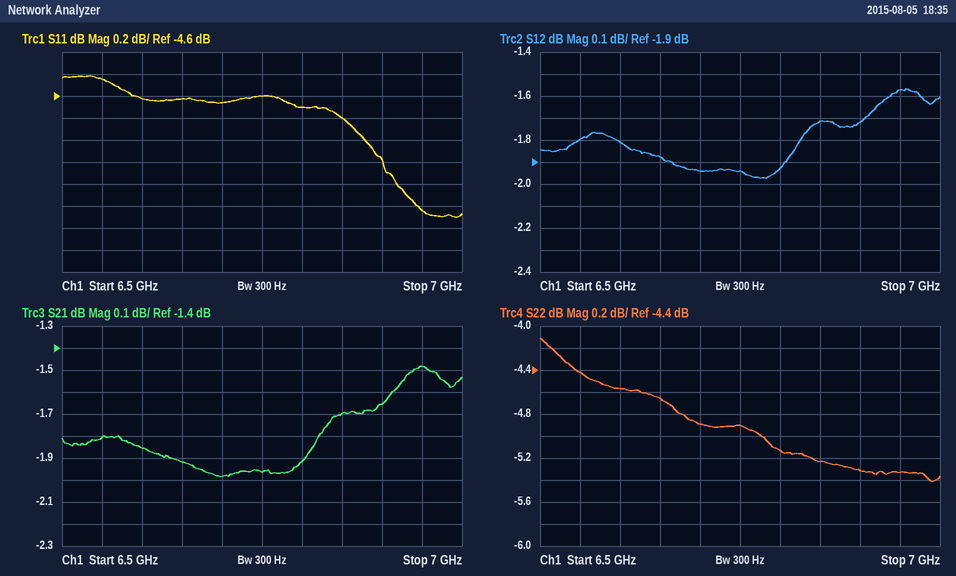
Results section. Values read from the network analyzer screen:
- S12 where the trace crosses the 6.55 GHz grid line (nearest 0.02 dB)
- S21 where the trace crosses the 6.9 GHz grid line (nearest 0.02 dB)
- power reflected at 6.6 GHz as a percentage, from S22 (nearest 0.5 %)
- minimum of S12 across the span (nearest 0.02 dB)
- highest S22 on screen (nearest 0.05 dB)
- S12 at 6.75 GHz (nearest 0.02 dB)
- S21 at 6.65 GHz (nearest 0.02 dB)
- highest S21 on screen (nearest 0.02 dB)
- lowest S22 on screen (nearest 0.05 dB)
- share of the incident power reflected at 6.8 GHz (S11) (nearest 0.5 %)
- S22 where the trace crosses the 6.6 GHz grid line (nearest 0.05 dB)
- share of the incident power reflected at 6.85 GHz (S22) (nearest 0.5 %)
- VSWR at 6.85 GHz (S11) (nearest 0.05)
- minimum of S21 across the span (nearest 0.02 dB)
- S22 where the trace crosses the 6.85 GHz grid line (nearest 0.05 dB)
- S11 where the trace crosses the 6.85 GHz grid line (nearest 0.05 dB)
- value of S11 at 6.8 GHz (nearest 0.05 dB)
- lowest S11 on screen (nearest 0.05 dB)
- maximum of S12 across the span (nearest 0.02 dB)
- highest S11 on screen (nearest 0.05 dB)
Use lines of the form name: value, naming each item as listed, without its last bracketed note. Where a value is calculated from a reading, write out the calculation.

S12 where the trace crosses the 6.55 GHz grid line: -1.80 dB
S21 where the trace crosses the 6.9 GHz grid line: -1.66 dB
power reflected at 6.6 GHz as a percentage, from S22: 10^(-4.55/10) ≈ 35.1 %, so 35.0 % to the nearest 0.5 %
minimum of S12 across the span: -1.98 dB
highest S22 on screen: -4.10 dB
S12 at 6.75 GHz: -1.94 dB
S21 at 6.65 GHz: -1.92 dB
highest S21 on screen: -1.48 dB
lowest S22 on screen: -5.40 dB
share of the incident power reflected at 6.8 GHz (S11): 10^(-4.7/10) ≈ 33.9 %, so 34.0 % to the nearest 0.5 %
S22 where the trace crosses the 6.6 GHz grid line: -4.55 dB
share of the incident power reflected at 6.85 GHz (S22): 10^(-5.25/10) ≈ 29.9 %, so 30.0 % to the nearest 0.5 %
VSWR at 6.85 GHz (S11): |Γ| = 10^(-4.8/20) = 0.5754; VSWR = (1 + 0.5754)/(1 − 0.5754) ≈ 3.71, so 3.70 to the nearest 0.05
minimum of S21 across the span: -1.98 dB
S22 where the trace crosses the 6.85 GHz grid line: -5.25 dB
S11 where the trace crosses the 6.85 GHz grid line: -4.80 dB
value of S11 at 6.8 GHz: -4.70 dB
lowest S11 on screen: -5.70 dB
maximum of S12 across the span: -1.56 dB
highest S11 on screen: -4.40 dB
